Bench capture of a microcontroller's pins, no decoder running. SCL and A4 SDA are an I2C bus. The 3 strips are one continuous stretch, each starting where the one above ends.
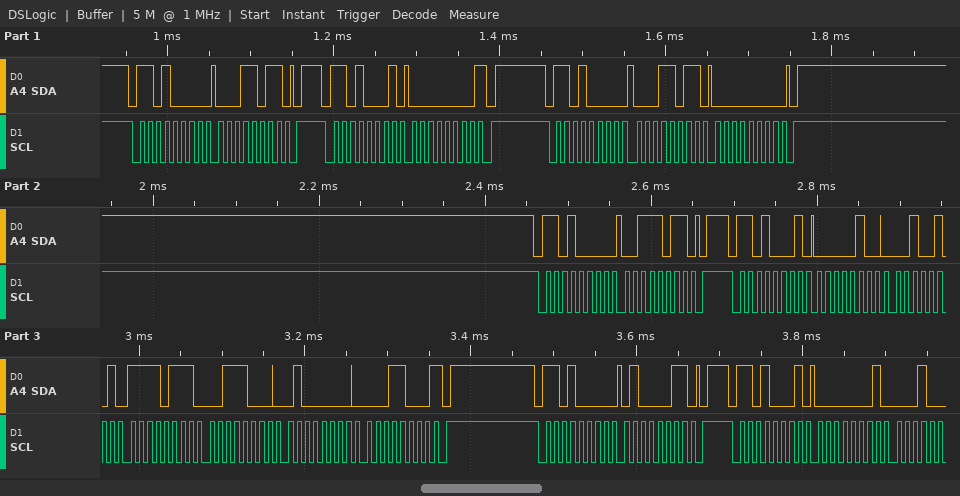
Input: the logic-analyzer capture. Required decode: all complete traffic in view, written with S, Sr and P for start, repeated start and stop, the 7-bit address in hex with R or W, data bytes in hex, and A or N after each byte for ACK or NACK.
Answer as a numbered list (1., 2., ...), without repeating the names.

1. S 68W A 1B A P S 68R A 00 N P S 68W A 1B A 00 A P S 68W A 3B A P S 68R A 04 A 25 A F7 A 38 A 40 A 18 N P S 68W A 43 A P S 68R A 01 A
